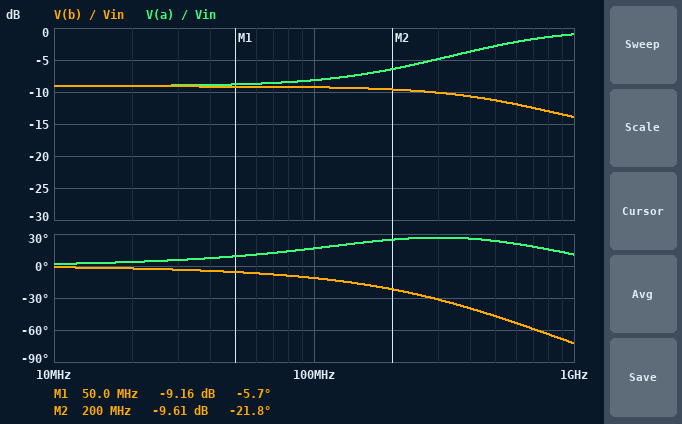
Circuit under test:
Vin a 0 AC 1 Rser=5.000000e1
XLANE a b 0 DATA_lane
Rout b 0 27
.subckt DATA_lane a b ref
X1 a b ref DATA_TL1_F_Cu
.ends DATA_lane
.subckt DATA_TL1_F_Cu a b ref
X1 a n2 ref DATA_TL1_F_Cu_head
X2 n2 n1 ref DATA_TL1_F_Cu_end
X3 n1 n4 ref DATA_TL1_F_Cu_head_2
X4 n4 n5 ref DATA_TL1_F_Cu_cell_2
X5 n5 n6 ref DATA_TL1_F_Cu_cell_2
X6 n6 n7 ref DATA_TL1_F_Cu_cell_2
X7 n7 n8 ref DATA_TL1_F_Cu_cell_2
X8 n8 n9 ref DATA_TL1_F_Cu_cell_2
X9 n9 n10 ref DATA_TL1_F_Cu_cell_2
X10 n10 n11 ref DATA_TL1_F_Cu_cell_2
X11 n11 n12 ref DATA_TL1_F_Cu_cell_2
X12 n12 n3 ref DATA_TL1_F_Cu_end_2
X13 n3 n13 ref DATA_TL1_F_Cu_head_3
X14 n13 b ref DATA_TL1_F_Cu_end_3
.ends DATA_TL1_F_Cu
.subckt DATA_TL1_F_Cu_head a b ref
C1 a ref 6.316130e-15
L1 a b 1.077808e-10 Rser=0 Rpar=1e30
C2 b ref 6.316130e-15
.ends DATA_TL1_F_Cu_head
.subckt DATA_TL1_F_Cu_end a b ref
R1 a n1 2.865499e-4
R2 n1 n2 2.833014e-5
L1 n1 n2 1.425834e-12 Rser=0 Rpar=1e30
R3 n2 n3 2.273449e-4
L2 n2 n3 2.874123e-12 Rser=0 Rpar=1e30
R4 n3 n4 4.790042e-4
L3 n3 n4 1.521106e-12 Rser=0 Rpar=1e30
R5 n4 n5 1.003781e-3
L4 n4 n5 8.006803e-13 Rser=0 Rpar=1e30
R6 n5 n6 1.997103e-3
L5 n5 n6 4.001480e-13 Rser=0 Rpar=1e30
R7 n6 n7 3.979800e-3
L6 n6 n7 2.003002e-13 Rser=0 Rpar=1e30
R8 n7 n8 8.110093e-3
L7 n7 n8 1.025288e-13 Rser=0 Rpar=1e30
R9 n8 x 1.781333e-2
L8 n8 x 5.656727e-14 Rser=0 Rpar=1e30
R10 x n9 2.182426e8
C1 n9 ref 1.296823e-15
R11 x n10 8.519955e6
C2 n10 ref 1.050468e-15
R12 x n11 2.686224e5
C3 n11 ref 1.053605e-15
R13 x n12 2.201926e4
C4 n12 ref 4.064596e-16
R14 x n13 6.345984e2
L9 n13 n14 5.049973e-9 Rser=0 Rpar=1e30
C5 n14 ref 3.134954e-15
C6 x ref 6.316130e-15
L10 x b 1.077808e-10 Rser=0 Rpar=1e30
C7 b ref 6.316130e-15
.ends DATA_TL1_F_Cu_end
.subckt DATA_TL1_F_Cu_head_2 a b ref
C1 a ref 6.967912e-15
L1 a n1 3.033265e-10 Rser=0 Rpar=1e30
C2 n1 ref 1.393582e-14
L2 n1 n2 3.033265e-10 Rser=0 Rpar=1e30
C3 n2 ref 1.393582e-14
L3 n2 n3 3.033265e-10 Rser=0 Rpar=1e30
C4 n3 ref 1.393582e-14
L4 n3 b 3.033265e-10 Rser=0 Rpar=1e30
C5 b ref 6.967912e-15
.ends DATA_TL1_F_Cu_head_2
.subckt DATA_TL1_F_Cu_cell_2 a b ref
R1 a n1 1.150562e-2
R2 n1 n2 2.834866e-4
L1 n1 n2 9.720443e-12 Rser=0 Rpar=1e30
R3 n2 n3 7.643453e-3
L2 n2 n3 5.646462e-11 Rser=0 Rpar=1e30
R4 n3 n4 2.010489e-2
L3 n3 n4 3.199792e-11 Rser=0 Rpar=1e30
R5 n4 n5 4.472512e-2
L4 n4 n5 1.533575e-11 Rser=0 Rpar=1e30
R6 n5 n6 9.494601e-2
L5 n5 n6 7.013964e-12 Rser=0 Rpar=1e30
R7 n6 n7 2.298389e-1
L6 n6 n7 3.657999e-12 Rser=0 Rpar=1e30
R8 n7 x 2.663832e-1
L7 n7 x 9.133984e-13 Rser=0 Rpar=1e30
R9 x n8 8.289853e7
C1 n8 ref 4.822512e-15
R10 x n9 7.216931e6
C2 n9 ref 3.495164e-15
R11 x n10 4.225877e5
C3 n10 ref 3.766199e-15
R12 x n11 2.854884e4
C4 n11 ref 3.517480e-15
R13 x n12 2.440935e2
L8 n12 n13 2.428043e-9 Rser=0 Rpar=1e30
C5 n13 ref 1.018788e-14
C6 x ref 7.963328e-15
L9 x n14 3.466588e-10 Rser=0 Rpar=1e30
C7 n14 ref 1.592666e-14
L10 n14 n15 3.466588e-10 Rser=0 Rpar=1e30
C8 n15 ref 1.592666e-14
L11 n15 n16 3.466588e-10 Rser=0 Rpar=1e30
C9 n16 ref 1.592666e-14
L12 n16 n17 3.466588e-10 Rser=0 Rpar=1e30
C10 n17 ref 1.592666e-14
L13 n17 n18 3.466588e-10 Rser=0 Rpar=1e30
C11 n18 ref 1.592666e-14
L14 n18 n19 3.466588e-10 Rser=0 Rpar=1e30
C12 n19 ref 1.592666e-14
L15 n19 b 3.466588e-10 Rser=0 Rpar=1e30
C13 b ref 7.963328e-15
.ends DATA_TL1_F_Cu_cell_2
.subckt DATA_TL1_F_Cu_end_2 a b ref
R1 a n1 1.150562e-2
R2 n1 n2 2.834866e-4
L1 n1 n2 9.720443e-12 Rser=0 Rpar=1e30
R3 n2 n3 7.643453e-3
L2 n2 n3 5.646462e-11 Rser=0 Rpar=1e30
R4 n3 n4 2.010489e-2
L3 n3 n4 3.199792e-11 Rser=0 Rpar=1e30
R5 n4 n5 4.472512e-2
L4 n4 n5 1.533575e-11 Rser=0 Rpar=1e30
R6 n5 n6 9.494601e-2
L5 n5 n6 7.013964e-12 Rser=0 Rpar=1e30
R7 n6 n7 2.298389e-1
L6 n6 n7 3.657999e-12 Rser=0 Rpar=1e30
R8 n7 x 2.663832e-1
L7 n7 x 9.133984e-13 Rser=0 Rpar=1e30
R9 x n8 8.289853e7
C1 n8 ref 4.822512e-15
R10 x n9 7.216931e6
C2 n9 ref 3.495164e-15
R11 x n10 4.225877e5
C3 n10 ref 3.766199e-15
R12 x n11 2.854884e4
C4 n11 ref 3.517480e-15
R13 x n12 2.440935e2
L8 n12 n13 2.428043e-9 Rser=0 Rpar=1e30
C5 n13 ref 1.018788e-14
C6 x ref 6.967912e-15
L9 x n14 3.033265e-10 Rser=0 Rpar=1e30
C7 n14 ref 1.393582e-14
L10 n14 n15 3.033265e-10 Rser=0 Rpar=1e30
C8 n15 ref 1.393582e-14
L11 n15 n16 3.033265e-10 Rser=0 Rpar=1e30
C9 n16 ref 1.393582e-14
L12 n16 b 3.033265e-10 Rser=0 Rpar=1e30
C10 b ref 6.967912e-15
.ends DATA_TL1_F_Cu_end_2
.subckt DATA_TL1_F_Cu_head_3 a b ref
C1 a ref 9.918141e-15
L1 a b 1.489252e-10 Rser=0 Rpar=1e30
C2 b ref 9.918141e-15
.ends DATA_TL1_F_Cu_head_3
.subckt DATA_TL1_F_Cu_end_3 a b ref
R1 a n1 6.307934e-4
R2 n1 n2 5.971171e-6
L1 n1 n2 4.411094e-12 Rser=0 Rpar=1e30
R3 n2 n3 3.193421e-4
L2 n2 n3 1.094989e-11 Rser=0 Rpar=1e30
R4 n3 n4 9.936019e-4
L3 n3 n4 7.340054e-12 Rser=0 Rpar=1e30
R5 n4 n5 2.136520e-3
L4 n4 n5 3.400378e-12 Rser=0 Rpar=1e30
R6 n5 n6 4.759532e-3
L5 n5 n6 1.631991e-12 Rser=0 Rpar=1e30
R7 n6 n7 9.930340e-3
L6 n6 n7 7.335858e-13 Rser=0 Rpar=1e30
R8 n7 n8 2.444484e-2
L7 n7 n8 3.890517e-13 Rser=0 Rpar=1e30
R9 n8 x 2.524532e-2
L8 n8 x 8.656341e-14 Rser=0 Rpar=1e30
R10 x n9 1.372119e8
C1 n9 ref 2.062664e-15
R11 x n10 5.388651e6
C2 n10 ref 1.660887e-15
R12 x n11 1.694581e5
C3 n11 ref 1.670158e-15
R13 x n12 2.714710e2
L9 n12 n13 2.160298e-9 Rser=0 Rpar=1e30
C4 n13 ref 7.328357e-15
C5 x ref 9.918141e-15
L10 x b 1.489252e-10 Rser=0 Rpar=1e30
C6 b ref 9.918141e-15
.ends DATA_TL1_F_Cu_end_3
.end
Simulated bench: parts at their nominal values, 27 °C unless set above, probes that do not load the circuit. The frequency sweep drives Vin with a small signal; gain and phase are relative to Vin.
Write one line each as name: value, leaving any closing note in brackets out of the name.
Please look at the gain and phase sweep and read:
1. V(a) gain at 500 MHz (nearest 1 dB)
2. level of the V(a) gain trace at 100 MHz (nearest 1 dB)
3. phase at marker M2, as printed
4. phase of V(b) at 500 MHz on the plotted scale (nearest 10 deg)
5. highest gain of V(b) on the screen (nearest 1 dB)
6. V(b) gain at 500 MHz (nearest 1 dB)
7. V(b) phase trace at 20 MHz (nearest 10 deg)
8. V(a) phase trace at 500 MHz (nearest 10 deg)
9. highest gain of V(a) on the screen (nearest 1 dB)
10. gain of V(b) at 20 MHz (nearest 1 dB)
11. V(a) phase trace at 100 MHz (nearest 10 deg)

V(a) gain at 500 MHz: -3 dB
level of the V(a) gain trace at 100 MHz: -8 dB
phase at marker M2, as printed: -21.8 deg
phase of V(b) at 500 MHz on the plotted scale: -50 deg
highest gain of V(b) on the screen: -9 dB
V(b) gain at 500 MHz: -11 dB
V(b) phase trace at 20 MHz: 0 deg
V(a) phase trace at 500 MHz: 20 deg
highest gain of V(a) on the screen: -1 dB
gain of V(b) at 20 MHz: -9 dB
V(a) phase trace at 100 MHz: 20 deg
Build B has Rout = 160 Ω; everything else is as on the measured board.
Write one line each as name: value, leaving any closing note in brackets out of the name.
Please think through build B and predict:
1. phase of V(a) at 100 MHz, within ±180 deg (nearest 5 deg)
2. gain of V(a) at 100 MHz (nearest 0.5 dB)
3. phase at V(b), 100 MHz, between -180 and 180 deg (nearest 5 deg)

phase of V(a) at 100 MHz, within ±180 deg: 0 deg
gain of V(a) at 100 MHz: -2.5 dB
phase at V(b), 100 MHz, between -180 and 180 deg: -5 deg
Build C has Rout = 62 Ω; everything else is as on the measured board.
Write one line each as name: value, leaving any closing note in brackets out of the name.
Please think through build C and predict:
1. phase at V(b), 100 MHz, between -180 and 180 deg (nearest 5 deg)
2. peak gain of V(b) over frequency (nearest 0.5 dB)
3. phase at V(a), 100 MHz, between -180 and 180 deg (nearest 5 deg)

phase at V(b), 100 MHz, between -180 and 180 deg: -10 deg
peak gain of V(b) over frequency: -5.0 dB
phase at V(a), 100 MHz, between -180 and 180 deg: 5 deg
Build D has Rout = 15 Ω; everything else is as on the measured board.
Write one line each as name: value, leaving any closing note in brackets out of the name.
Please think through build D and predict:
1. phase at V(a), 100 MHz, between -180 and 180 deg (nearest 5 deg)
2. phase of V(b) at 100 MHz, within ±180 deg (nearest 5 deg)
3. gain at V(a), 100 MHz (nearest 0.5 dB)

phase at V(a), 100 MHz, between -180 and 180 deg: 30 deg
phase of V(b) at 100 MHz, within ±180 deg: -15 deg
gain at V(a), 100 MHz: -10.0 dB
